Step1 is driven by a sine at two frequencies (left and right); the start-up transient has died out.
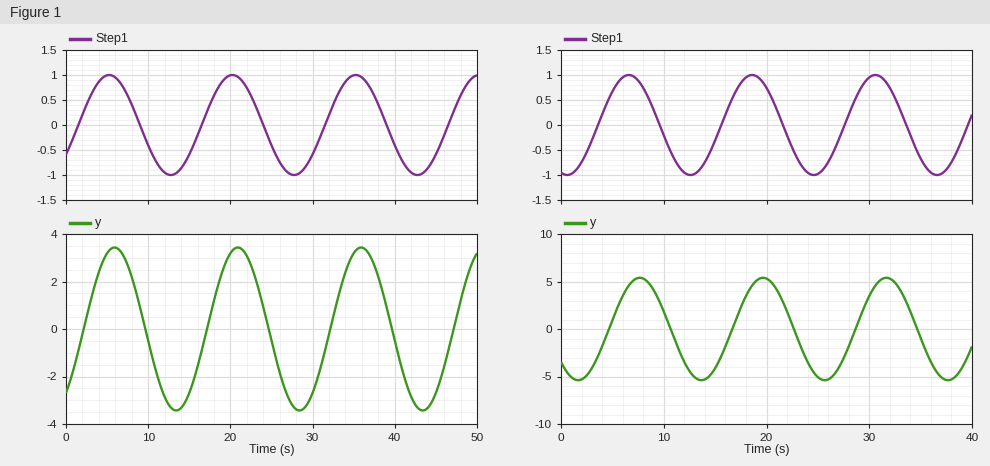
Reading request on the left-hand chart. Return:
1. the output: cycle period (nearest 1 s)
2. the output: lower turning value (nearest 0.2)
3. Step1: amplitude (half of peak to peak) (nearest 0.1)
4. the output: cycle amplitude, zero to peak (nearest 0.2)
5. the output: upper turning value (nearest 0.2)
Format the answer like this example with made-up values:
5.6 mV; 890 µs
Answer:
15 s; -3.4; 1.0; 3.4; 3.4
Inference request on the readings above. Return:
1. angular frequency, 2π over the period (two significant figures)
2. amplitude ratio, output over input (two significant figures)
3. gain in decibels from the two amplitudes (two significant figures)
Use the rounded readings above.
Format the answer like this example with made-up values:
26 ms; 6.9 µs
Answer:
0.42 rad/s; 3.4; 11 dB
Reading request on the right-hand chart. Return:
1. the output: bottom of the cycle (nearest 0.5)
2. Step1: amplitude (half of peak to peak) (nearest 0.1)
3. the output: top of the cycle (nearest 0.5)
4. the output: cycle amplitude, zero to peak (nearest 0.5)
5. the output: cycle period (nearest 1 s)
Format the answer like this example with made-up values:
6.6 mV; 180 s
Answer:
-5.5; 1.0; 5.5; 5.5; 12 s
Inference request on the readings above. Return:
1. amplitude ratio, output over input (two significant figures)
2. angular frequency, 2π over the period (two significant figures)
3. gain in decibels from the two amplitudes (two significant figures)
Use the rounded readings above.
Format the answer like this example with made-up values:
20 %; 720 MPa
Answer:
5.5; 0.52 rad/s; 15 dB
